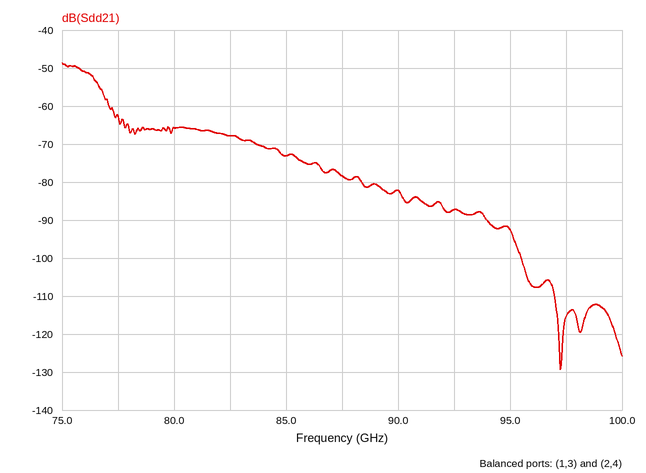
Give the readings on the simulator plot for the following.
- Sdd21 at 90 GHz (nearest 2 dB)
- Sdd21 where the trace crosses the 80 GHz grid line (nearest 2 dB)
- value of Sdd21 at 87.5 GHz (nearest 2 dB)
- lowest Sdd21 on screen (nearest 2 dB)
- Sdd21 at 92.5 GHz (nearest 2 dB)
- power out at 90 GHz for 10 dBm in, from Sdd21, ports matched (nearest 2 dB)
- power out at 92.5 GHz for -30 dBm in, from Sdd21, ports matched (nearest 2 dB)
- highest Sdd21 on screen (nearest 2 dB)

-82 dB
-66 dB
-78 dB
-130 dB
-88 dB
-72 dBm
-118 dBm
-48 dB
